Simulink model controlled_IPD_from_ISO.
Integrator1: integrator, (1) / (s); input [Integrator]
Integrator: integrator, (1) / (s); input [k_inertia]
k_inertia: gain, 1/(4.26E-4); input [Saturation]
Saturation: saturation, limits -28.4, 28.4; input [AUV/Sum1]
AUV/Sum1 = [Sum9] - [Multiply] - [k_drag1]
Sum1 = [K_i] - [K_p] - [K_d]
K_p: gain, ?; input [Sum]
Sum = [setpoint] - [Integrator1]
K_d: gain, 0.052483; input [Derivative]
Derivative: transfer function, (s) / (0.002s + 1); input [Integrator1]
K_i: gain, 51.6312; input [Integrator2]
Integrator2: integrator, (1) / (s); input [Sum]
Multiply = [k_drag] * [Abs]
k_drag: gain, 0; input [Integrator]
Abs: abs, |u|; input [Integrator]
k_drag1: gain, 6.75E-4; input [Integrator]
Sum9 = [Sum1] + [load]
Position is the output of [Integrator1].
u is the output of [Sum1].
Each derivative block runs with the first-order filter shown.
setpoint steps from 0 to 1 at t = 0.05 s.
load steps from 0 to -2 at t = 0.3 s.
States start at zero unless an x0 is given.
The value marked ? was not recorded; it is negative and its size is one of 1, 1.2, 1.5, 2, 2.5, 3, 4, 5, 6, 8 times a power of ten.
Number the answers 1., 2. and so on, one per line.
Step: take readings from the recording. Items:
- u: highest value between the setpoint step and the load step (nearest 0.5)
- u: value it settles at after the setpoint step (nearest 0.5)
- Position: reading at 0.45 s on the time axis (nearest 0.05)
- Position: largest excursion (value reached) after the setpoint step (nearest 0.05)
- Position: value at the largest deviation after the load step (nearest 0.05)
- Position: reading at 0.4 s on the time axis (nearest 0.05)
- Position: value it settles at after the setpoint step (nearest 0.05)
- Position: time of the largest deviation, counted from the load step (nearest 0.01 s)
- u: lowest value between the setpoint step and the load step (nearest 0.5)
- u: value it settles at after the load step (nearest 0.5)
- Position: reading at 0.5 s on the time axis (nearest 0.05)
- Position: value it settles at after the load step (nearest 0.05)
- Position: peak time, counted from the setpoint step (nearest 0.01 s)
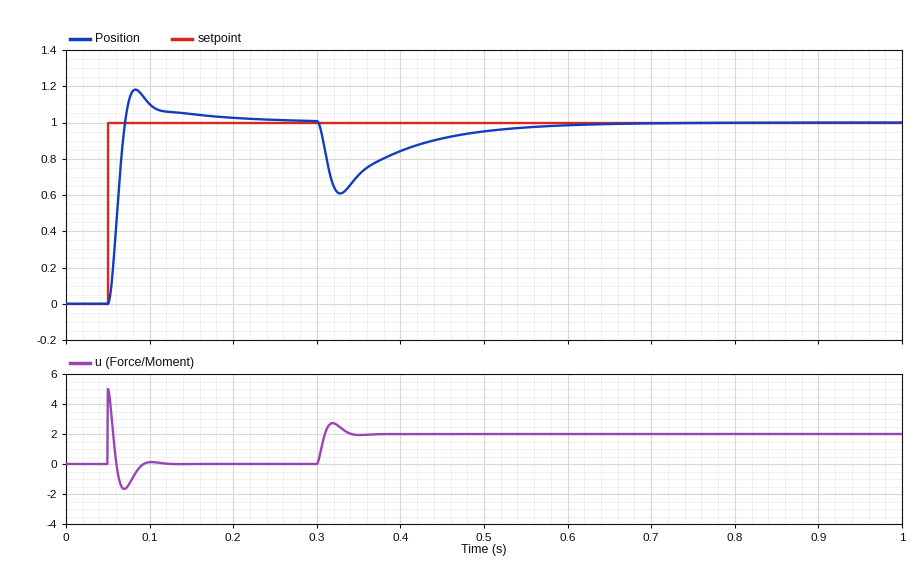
1. 5.0
2. 0.0
3. 0.90
4. 1.20
5. 0.60
6. 0.85
7. 1.00
8. 0.03 s
9. -1.5
10. 2.0
11. 0.95
12. 1.00
13. 0.03 s
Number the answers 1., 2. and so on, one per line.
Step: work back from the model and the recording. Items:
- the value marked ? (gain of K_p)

1. -5
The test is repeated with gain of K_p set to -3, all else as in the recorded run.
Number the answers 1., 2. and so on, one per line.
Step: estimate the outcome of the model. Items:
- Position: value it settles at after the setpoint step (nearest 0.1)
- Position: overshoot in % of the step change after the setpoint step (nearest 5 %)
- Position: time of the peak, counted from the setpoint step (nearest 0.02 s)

1. 1.0
2. 25 %
3. 0.06 s
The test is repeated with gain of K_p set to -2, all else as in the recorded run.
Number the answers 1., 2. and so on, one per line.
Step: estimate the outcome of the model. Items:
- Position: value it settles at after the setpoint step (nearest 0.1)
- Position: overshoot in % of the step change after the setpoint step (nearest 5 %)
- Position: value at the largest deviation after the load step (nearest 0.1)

1. 1.0
2. 35 %
3. 0.3
